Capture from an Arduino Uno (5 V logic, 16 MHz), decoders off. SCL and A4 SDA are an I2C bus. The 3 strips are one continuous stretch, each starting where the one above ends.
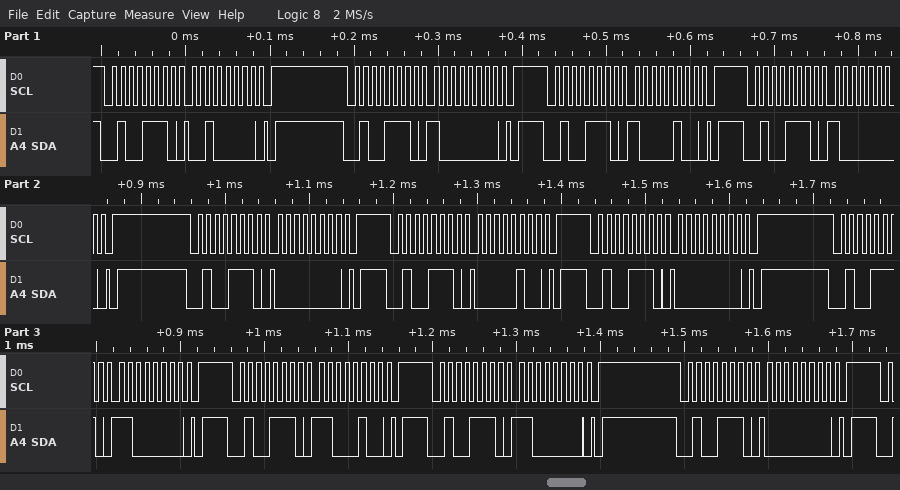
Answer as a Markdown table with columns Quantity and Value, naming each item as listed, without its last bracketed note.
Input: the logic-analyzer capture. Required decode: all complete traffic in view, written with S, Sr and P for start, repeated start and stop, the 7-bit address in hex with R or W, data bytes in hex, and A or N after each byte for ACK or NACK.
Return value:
| Quantity | Value |
|---|---|
| all complete traffic in view, written with S, Sr and P for start, repeated start and stop, the 7-bit address in hex with R or W, data bytes in hex, and A or N after each byte for ACK or NACK | S 27W A 20 A P S 27W A 80 A P S 27W A 84 A P S 27W A 80 A P S 27W A 00 A P S 27W A 04 A P S 27W A 00 A P S 27W A C0 A P S 27W A C4 A P S 27W A C0 A P S 27W A 00 A P |
